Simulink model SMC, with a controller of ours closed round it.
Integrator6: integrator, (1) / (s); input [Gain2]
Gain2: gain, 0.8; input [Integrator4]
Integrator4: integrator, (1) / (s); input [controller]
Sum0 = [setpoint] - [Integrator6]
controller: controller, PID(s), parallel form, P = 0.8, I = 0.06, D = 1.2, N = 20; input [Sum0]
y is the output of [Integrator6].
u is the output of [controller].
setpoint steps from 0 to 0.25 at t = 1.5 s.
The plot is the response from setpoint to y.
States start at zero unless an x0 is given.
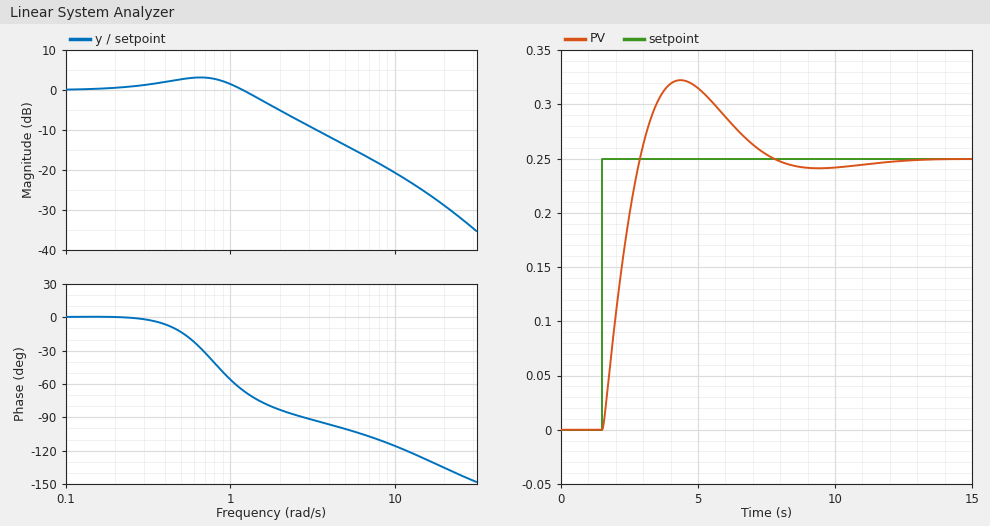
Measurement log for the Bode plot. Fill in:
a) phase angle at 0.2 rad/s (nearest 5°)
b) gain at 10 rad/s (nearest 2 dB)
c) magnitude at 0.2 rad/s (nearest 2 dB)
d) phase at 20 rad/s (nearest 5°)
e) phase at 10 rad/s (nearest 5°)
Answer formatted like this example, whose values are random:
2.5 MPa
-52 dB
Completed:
0°
-20 dB
0 dB
-135°
-115°
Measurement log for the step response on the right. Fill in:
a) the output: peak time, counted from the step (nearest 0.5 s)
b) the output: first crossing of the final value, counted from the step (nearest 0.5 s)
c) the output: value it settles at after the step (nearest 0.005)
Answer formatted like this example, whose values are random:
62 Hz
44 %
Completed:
3.0 s
1.5 s
0.250
